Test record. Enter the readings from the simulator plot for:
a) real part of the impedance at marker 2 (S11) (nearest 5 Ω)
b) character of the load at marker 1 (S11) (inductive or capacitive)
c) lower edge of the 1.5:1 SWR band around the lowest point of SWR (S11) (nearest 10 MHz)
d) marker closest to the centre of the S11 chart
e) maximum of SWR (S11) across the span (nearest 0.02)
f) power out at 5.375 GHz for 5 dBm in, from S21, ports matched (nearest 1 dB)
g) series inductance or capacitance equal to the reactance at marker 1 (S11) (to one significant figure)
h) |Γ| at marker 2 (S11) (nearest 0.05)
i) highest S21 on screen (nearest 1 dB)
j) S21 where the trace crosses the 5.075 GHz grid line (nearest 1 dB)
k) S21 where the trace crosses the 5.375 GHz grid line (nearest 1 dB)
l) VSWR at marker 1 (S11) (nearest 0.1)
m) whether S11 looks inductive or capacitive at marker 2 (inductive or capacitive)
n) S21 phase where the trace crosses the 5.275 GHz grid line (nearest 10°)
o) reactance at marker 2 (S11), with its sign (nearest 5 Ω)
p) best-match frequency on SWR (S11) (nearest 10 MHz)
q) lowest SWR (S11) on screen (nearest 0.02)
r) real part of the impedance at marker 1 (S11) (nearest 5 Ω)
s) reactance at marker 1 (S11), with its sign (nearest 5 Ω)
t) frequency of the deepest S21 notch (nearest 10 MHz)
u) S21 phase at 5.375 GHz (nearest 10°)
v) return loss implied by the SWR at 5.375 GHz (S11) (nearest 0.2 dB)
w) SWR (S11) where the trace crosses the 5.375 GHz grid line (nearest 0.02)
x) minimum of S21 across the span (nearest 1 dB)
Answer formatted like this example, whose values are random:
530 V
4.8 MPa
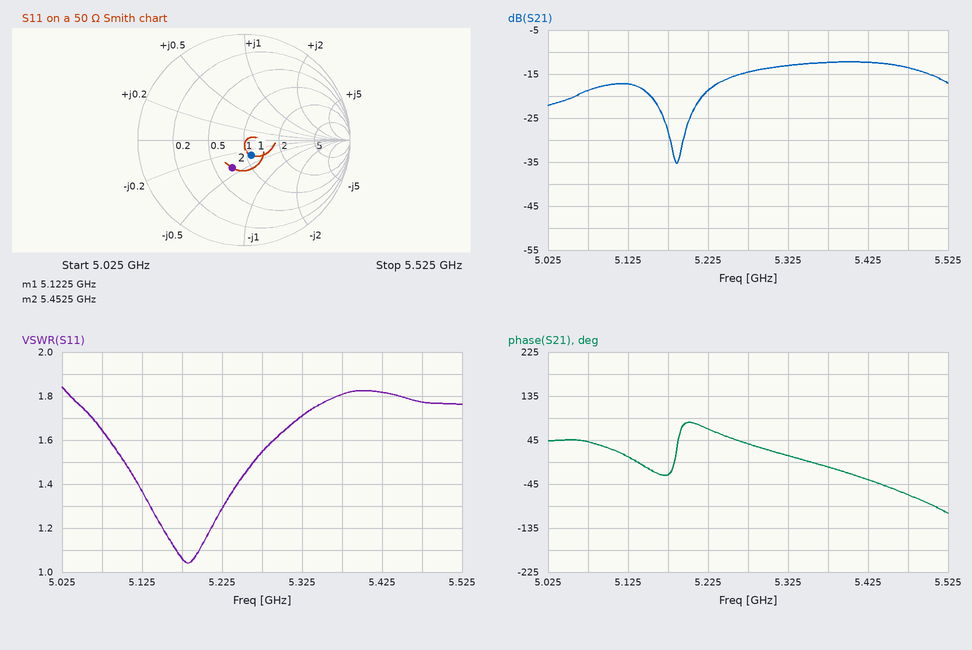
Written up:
35 Ω
capacitive
5.10 GHz
marker 1
1.84
-7 dBm
2 pF
0.30
-12 dB
-19 dB
-12 dB
1.4
capacitive
40°
-20 Ω
5.18 GHz
1.04
55 Ω
-15 Ω
5.19 GHz
-10°
10.8 dB
1.80
-35 dB
